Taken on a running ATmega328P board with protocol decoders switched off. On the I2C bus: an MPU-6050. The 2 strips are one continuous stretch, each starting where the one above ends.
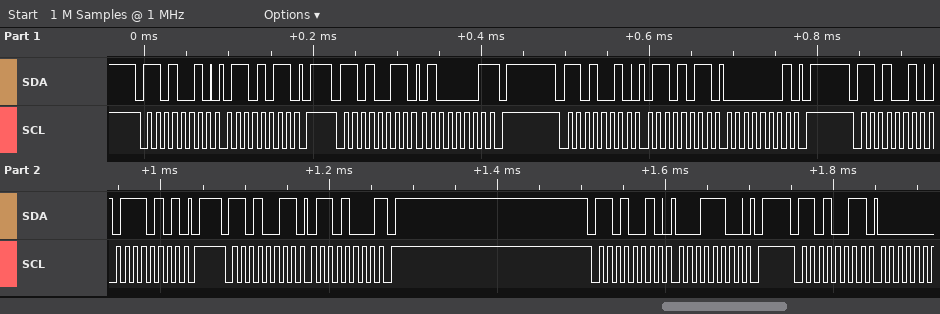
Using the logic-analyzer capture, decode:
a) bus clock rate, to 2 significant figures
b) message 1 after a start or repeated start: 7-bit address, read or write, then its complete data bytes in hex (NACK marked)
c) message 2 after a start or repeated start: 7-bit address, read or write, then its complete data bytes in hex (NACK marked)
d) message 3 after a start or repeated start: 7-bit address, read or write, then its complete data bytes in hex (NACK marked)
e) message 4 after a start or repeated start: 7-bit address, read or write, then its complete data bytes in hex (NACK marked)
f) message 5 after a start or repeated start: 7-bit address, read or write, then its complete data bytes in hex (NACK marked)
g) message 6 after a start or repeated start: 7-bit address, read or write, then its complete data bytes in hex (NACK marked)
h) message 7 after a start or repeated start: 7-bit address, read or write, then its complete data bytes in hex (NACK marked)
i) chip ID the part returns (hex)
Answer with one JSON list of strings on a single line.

["100 kHz", "0x69 write: 6B", "0x69 read: 41 NACK", "0x69 write: 6B 01", "0x69 write: 75", "0x69 read: 68 NACK", "0x69 write: 1C", "0x69 read", "0x68"]
